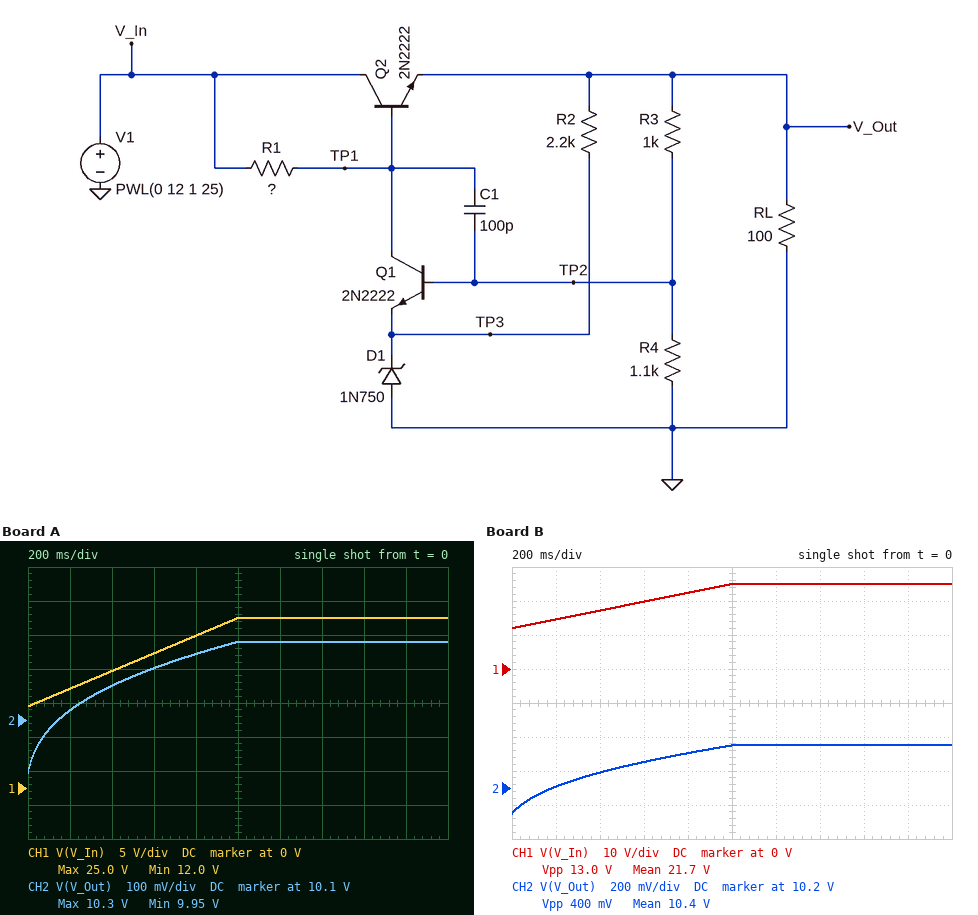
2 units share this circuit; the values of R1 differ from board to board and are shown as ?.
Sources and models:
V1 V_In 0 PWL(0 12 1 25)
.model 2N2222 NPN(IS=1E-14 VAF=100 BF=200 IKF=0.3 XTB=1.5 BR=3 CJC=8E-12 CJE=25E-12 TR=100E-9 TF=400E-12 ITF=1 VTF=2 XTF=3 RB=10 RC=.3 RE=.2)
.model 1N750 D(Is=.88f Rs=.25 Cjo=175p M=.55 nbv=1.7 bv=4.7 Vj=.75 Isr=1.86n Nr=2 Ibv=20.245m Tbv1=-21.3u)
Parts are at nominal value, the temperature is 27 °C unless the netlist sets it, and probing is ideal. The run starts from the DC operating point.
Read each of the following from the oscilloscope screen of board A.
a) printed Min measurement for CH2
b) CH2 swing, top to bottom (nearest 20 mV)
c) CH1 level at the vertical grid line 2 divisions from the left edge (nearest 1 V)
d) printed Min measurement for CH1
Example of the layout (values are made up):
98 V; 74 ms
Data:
9.95 V; 380 mV; 17 V; 12.0 V
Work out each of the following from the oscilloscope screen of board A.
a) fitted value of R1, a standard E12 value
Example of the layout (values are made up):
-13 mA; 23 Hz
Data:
1.5 kΩ
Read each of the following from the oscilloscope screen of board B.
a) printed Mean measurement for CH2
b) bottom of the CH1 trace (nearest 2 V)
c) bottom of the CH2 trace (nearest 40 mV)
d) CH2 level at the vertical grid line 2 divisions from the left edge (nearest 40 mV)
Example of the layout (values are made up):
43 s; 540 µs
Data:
10.4 V; 12 V; 10.04 V; 10.28 V
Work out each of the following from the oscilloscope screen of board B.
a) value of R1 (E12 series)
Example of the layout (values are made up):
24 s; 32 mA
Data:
820 Ω
